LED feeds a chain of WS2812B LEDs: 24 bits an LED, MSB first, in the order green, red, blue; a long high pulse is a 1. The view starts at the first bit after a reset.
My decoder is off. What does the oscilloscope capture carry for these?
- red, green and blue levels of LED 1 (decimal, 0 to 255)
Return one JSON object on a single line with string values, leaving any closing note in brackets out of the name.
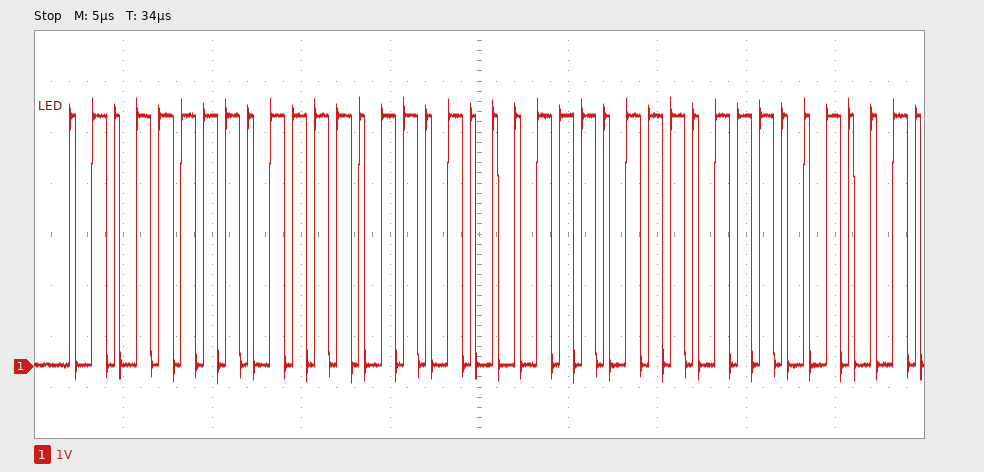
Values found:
{"red, green and blue levels of LED 1": "123, 95, 71"}
